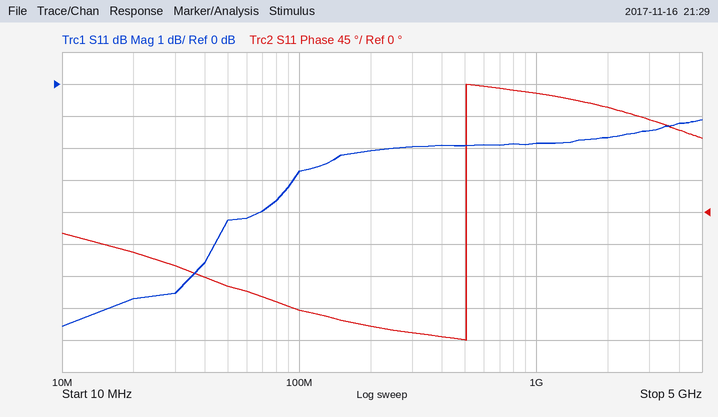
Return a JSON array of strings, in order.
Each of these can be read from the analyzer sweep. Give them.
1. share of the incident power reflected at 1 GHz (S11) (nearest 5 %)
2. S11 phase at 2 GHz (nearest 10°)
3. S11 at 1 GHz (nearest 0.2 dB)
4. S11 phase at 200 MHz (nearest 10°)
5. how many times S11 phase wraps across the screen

["65 %", "150°", "-1.8 dB", "-160°", "1"]
